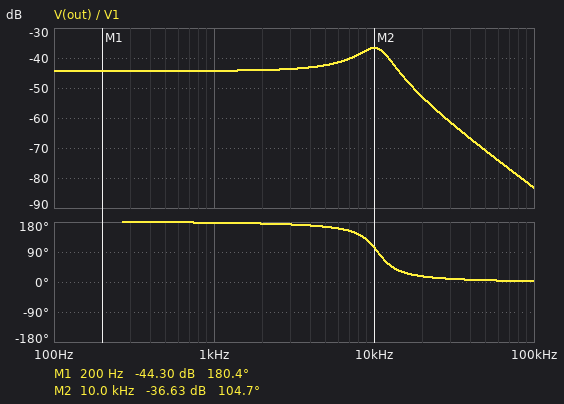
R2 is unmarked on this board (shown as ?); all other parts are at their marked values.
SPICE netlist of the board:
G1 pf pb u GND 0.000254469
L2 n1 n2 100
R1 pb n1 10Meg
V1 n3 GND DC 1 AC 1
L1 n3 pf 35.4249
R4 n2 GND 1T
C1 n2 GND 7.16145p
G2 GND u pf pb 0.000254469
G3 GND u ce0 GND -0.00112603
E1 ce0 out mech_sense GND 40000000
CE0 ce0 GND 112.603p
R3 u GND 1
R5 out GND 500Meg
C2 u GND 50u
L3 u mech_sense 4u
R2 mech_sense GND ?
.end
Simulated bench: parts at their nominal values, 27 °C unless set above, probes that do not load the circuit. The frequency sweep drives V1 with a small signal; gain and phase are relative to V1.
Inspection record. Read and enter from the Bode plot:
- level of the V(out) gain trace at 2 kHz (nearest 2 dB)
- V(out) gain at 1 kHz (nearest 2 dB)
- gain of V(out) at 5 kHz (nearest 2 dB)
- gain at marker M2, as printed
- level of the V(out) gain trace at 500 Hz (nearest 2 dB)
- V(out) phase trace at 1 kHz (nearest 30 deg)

-44 dB
-44 dB
-42 dB
-36.63 dB
-44 dB
180 deg
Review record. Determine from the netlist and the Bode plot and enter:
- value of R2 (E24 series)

620 nΩ
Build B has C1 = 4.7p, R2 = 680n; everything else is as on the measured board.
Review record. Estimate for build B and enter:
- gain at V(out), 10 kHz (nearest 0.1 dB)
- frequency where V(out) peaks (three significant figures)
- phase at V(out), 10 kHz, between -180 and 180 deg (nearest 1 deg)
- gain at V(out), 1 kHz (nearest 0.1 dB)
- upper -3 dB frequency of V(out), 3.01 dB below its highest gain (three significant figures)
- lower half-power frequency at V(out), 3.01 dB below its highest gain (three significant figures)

-35.9 dB
10.2 kHz
107 deg
-43.6 dB
12.3 kHz
7.56 kHz
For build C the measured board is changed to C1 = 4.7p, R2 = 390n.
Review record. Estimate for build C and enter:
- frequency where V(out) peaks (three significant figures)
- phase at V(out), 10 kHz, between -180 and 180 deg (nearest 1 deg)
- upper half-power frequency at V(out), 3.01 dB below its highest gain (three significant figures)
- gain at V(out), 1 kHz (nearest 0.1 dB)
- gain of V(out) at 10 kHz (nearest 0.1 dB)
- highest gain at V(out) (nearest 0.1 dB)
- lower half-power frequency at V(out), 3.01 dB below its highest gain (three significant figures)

10.2 kHz
107 deg
12.3 kHz
-48.4 dB
-40.8 dB
-40.7 dB
7.56 kHz
